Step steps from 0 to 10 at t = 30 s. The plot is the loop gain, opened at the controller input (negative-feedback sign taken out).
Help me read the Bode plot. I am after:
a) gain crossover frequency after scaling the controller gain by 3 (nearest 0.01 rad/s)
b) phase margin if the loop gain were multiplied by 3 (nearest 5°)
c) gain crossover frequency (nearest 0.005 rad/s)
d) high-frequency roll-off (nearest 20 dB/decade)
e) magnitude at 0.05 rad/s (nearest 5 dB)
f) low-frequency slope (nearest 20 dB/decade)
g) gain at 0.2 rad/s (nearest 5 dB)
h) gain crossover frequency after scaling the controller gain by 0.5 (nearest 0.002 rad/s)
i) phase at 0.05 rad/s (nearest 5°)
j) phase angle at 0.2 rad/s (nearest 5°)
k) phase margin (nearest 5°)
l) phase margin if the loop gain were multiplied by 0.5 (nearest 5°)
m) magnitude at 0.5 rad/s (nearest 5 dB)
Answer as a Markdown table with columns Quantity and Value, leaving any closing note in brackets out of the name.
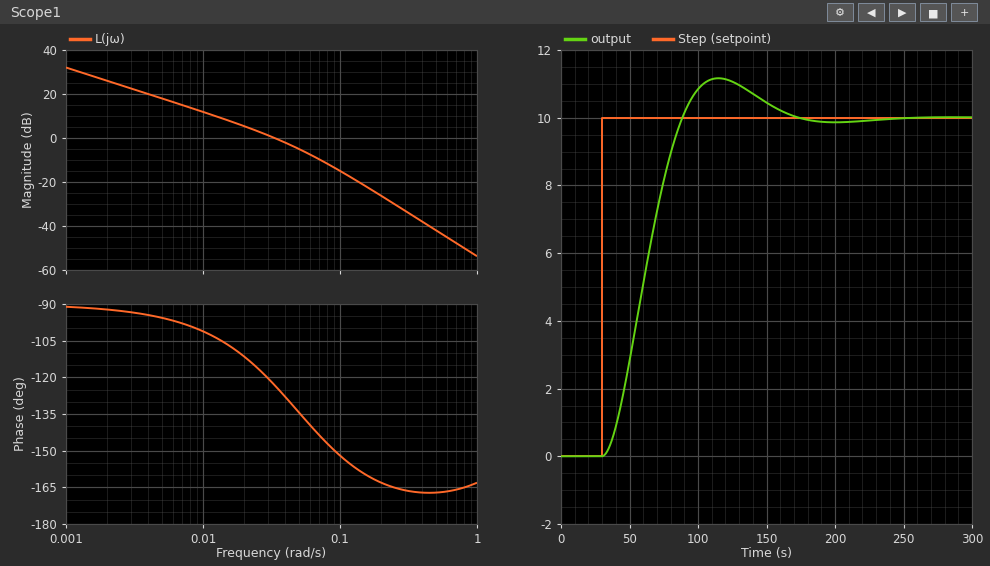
| Quantity | Value |
|---|---|
| gain crossover frequency after scaling the controller gain by 3 | 0.07 rad/s |
| phase margin if the loop gain were multiplied by 3 | 35° |
| gain crossover frequency | 0.035 rad/s |
| high-frequency roll-off | -40 dB/decade |
| magnitude at 0.05 rad/s | -5 dB |
| low-frequency slope | -20 dB/decade |
| gain at 0.2 rad/s | -25 dB |
| gain crossover frequency after scaling the controller gain by 0.5 | 0.018 rad/s |
| phase at 0.05 rad/s | -135° |
| phase angle at 0.2 rad/s | -165° |
| phase margin | 55° |
| phase margin if the loop gain were multiplied by 0.5 | 70° |
| magnitude at 0.5 rad/s | -40 dB |
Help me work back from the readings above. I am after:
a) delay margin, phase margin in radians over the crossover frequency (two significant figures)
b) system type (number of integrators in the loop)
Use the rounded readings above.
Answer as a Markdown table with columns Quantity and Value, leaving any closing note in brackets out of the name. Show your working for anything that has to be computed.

| Quantity | Value |
|---|---|
| delay margin, phase margin in radians over the crossover frequency | 55 × π / 180 / 0.035 = 27 s |
| system type | 1 |
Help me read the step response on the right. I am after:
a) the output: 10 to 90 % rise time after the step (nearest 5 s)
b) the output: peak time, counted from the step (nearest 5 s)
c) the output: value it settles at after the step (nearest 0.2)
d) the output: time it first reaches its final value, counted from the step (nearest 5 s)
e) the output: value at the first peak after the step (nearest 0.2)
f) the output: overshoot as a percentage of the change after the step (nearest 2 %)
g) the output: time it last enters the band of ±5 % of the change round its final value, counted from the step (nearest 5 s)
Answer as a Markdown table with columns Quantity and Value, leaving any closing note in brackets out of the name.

| Quantity | Value |
|---|---|
| the output: 10 to 90 % rise time after the step | 40 s |
| the output: peak time, counted from the step | 85 s |
| the output: value it settles at after the step | 10.0 |
| the output: time it first reaches its final value, counted from the step | 60 s |
| the output: value at the first peak after the step | 11.2 |
| the output: overshoot as a percentage of the change after the step | 12 % |
| the output: time it last enters the band of ±5 % of the change round its final value, counted from the step | 120 s |
